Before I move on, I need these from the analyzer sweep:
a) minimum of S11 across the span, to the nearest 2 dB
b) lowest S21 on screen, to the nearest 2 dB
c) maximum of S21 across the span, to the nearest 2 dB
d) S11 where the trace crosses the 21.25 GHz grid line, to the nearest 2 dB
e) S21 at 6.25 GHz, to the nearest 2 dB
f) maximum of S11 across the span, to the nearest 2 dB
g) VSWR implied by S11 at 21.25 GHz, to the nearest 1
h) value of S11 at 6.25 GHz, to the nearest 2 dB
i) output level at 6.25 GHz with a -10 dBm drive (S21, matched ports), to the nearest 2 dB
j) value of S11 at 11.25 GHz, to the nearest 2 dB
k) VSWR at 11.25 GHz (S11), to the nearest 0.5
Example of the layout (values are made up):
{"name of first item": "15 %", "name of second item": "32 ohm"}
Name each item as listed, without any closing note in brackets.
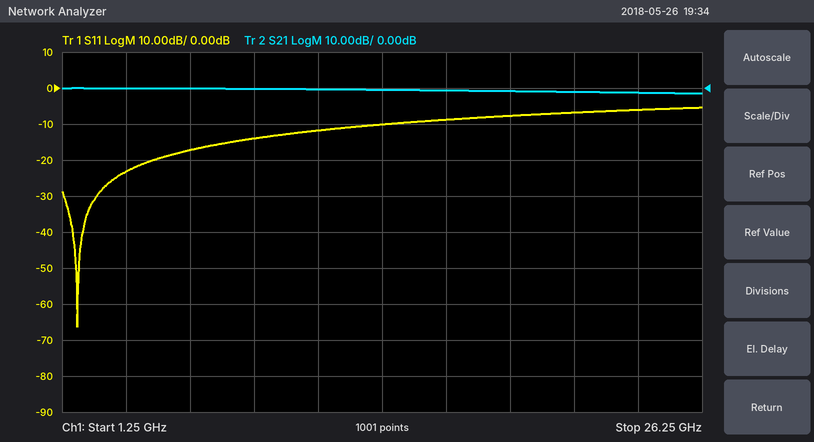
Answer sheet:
{"minimum of S11 across the span, to the nearest 2 dB": "-66 dB", "lowest S21 on screen, to the nearest 2 dB": "-2 dB", "maximum of S21 across the span, to the nearest 2 dB": "0 dB", "S11 where the trace crosses the 21.25 GHz grid line, to the nearest 2 dB": "-6 dB", "S21 at 6.25 GHz, to the nearest 2 dB": "0 dB", "maximum of S11 across the span, to the nearest 2 dB": "-6 dB", "VSWR implied by S11 at 21.25 GHz, to the nearest 1": "3", "value of S11 at 6.25 GHz, to the nearest 2 dB": "-18 dB", "output level at 6.25 GHz with a -10 dBm drive (S21, matched ports), to the nearest 2 dB": "-10 dBm", "value of S11 at 11.25 GHz, to the nearest 2 dB": "-12 dB", "VSWR at 11.25 GHz (S11), to the nearest 0.5": "1.5"}
